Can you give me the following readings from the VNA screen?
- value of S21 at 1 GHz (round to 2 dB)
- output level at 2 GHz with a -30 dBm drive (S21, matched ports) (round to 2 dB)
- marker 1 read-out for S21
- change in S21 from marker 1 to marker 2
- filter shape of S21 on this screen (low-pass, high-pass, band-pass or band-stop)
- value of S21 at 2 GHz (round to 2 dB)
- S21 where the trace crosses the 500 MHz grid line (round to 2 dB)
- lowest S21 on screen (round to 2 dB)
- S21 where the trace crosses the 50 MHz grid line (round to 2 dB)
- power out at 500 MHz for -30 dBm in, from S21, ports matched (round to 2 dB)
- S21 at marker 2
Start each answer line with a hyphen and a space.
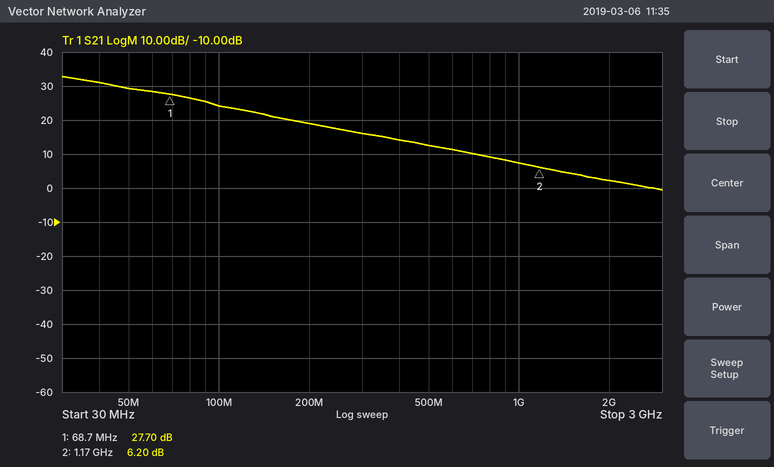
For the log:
- 8 dB
- -28 dBm
- 27.70 dB
- -21.50 dB
- low-pass
- 2 dB
- 12 dB
- 0 dB
- 30 dB
- -18 dBm
- 6.20 dB
